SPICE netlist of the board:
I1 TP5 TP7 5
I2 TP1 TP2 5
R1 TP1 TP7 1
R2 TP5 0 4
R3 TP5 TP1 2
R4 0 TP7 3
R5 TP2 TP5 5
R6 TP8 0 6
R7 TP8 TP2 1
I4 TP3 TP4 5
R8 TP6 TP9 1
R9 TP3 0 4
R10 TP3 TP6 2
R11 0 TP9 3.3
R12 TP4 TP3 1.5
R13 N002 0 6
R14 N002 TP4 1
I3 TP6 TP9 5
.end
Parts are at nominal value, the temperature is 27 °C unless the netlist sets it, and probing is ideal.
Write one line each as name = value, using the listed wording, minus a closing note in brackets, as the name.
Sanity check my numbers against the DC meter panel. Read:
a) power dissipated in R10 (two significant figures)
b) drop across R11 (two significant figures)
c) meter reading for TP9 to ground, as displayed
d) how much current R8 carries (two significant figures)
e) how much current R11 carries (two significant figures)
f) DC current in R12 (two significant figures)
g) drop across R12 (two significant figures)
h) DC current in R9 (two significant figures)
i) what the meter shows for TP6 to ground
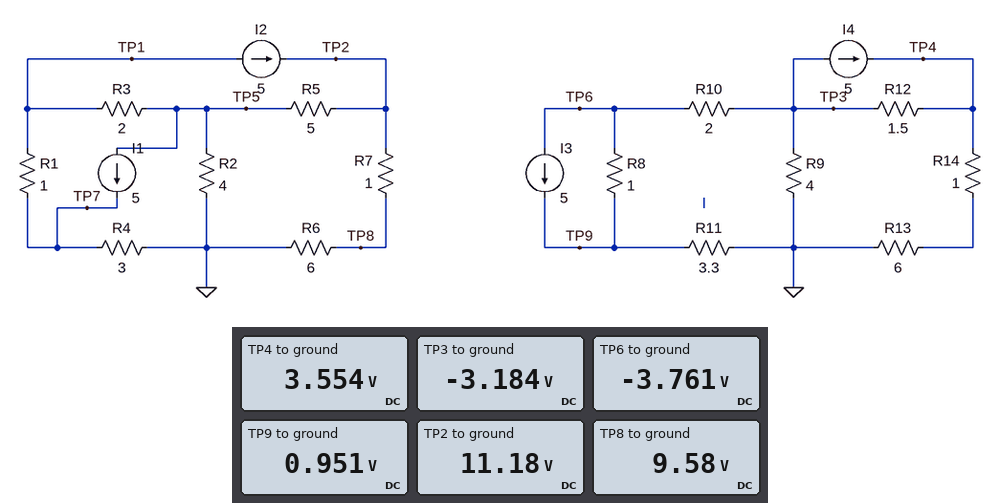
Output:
power dissipated in R10 = 170 mW
drop across R11 = 950 mV
meter reading for TP9 to ground, as displayed = 0.951 V
how much current R8 carries = 4.7 A
how much current R11 carries = 290 mA
DC current in R12 = 4.5 A
drop across R12 = 6.7 V
DC current in R9 = 800 mA
what the meter shows for TP6 to ground = -3.761 V
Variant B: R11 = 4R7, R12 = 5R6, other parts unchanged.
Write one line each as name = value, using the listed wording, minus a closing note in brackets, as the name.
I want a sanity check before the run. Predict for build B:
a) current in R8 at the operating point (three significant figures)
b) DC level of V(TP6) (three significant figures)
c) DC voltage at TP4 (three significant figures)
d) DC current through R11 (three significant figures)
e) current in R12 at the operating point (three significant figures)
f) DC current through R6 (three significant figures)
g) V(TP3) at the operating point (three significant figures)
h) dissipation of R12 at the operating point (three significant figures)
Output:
current in R8 at the operating point = 5.16 A
DC level of V(TP6) = -5.93 V
DC voltage at TP4 = 12.1 V
DC current through R11 = 163 mA
current in R12 at the operating point = 3.27 A
DC current through R6 = 1.60 A
V(TP3) at the operating point = -6.25 V
dissipation of R12 at the operating point = 60.0 W
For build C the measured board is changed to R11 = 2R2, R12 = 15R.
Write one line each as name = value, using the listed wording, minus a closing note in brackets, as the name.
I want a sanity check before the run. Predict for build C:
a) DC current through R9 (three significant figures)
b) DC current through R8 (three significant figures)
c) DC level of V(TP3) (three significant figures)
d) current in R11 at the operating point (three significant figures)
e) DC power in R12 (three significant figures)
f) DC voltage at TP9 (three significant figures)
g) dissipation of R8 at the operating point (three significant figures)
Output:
DC current through R9 = 2.24 A
DC current through R8 = 5.76 A
DC level of V(TP3) = -8.96 V
current in R11 at the operating point = 762 mA
DC power in R12 = 59.9 W
DC voltage at TP9 = -1.68 V
dissipation of R8 at the operating point = 33.2 W
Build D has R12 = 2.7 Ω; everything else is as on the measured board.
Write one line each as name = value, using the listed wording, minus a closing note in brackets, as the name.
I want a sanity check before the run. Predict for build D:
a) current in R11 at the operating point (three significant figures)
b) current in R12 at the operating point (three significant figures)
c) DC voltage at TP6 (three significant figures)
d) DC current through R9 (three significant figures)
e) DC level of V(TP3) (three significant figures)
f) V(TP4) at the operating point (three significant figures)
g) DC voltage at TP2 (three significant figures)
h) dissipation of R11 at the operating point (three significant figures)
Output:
current in R11 at the operating point = 116 mA
current in R12 at the operating point = 4.05 A
DC voltage at TP6 = -4.50 V
DC current through R9 = 1.07 A
DC level of V(TP3) = -4.27 V
V(TP4) at the operating point = 6.66 V
DC voltage at TP2 = 11.2 V
dissipation of R11 at the operating point = 44.3 mW
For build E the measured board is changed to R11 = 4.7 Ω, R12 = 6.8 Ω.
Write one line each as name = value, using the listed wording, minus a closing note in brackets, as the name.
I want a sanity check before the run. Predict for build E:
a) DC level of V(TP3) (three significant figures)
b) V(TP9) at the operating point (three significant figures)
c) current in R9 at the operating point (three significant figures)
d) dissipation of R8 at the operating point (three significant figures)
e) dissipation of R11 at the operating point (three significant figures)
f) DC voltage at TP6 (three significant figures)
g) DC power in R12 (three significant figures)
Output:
DC level of V(TP3) = -6.88 V
V(TP9) at the operating point = -1.15 V
current in R9 at the operating point = 1.72 A
dissipation of R8 at the operating point = 27.5 W
dissipation of R11 at the operating point = 281 mW
DC voltage at TP6 = -6.39 V
DC power in R12 = 62.6 W
